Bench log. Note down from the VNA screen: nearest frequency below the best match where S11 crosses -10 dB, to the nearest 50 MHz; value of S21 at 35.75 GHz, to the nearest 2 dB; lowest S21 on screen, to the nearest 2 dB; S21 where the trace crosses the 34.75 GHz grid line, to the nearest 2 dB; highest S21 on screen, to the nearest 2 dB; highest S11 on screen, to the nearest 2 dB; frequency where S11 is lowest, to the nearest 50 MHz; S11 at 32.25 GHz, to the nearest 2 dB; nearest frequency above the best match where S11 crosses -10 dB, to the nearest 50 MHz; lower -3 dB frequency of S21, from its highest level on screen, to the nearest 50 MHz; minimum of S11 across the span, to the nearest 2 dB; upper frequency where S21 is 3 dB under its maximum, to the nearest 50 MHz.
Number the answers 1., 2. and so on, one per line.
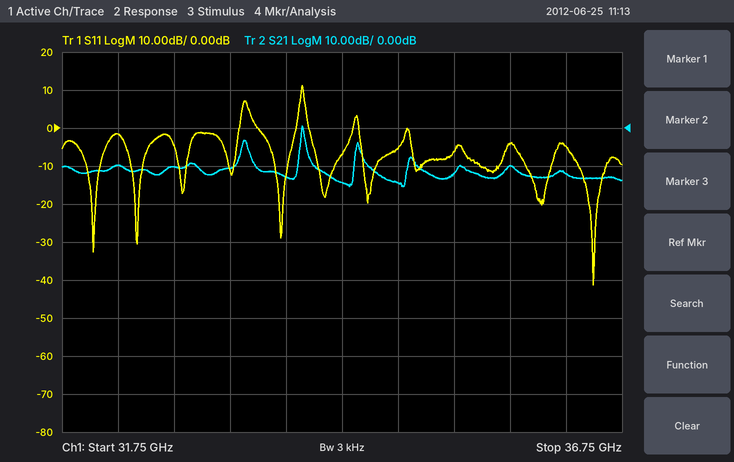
1. 36.35 GHz
2. -10 dB
3. -16 dB
4. -14 dB
5. 0 dB
6. 12 dB
7. 36.50 GHz
8. -2 dB
9. 36.60 GHz
10. 33.90 GHz
11. -42 dB
12. 33.90 GHz
